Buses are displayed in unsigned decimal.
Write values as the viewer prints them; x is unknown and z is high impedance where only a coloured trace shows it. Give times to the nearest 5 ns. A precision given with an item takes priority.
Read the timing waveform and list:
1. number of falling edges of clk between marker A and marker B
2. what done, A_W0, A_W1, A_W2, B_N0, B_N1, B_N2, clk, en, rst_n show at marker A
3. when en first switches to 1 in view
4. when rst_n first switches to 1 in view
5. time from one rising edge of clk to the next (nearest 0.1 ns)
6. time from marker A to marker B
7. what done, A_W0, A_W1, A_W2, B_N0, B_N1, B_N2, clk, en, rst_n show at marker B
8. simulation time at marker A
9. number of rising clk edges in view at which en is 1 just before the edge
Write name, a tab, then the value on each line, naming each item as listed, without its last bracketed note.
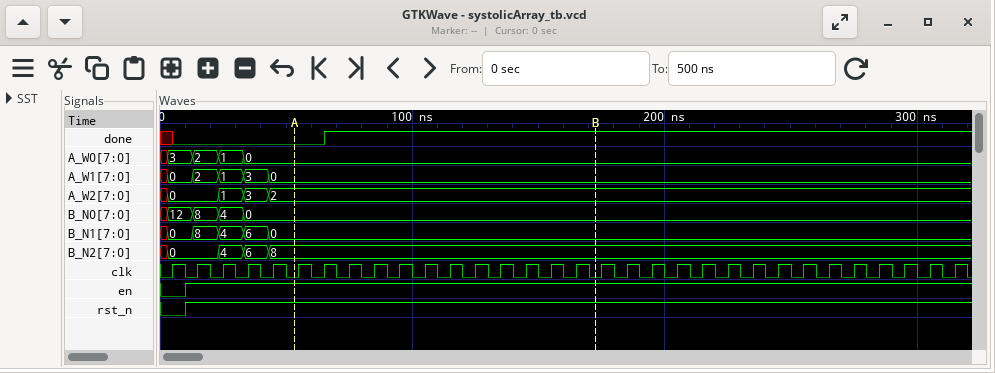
number of falling edges of clk between marker A and marker B	12
what done, A_W0, A_W1, A_W2, B_N0, B_N1, B_N2, clk, en, rst_n show at marker A	done=0, A_W0=0, A_W1=0, A_W2=2, B_N0=0, B_N1=0, B_N2=8, clk=0, en=1, rst_n=1
when en first switches to 1 in view	10 ns
when rst_n first switches to 1 in view	10 ns
time from one rising edge of clk to the next	10 ns
time from marker A to marker B	120 ns
what done, A_W0, A_W1, A_W2, B_N0, B_N1, B_N2, clk, en, rst_n show at marker B	done=1, A_W0=0, A_W1=0, A_W2=2, B_N0=0, B_N1=0, B_N2=8, clk=0, en=1, rst_n=1
simulation time at marker A	55 ns
number of rising clk edges in view at which en is 1 just before the edge	31
